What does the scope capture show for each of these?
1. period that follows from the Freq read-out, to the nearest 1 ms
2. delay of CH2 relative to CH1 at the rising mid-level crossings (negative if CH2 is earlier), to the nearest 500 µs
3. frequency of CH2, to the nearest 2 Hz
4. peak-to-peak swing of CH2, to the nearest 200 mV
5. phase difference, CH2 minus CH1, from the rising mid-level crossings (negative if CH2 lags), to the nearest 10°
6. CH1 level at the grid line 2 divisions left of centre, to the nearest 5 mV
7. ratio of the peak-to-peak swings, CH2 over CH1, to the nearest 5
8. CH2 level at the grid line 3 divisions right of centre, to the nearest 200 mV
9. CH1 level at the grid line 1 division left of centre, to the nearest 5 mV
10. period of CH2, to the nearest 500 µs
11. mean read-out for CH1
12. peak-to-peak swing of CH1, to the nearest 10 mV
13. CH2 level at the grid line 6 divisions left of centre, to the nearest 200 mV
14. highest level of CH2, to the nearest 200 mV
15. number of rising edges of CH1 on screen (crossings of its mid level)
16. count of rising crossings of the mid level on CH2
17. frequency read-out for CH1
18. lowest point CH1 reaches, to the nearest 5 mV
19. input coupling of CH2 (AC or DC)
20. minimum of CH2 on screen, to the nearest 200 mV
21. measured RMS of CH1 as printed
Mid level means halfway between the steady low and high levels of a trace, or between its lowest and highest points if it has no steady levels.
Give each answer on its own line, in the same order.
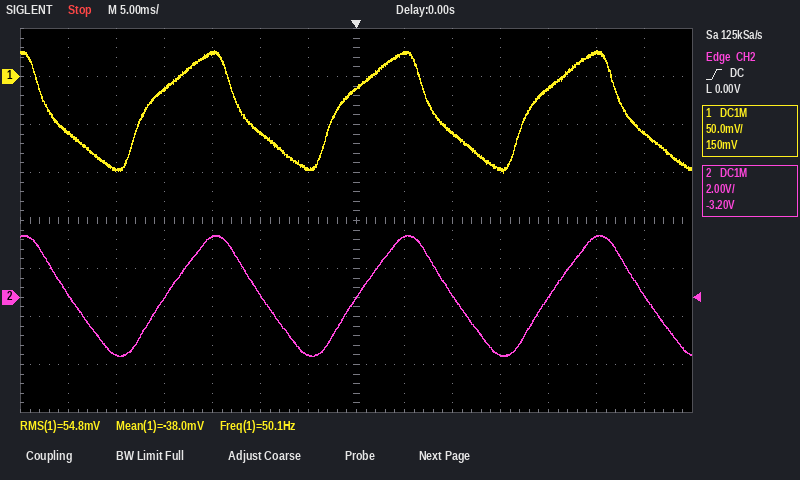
20 ms
+2.0 ms
50 Hz
5.0 V
-40°
-60 mV
40
-2.4 V
-95 mV
20.0 ms
-38.0 mV
130 mV
200 mV
2.6 V
3
3
50.1 Hz
-100 mV
DC
-2.4 V
54.8 mV
